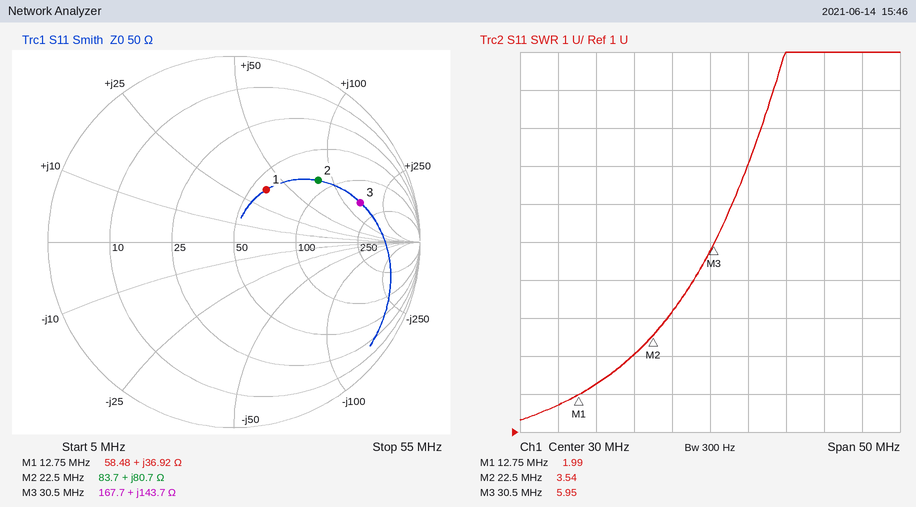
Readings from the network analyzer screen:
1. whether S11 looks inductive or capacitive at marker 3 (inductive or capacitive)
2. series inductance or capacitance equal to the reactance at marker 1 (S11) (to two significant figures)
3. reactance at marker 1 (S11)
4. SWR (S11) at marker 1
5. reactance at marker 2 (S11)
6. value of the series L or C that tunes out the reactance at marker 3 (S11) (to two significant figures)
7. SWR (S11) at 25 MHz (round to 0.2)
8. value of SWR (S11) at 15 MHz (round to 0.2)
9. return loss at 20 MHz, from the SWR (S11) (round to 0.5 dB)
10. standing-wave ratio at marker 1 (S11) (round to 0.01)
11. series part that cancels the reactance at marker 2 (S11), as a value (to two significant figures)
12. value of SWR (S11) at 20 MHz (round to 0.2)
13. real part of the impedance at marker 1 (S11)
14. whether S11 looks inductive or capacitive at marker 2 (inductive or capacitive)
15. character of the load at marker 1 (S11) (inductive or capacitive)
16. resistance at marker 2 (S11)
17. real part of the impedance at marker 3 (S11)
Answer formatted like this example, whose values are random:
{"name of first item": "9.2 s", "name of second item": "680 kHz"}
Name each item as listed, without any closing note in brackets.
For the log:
{"whether S11 looks inductive or capacitive at marker 3": "inductive", "series inductance or capacitance equal to the reactance at marker 1 (S11)": "460 nH", "reactance at marker 1": "+36.92 Ω", "SWR (S11) at marker 1": "1.99", "reactance at marker 2": "+80.7 Ω", "value of the series L or C that tunes out the reactance at marker 3 (S11)": "36 pF", "SWR (S11) at 25 MHz": "4.2", "value of SWR (S11) at 15 MHz": "2.2", "return loss at 20 MHz, from the SWR (S11)": "6.0 dB", "standing-wave ratio at marker 1 (S11)": "1.99", "series part that cancels the reactance at marker 2 (S11), as a value": "88 pF", "value of SWR (S11) at 20 MHz": "3.0", "real part of the impedance at marker 1": "58.48 Ω", "whether S11 looks inductive or capacitive at marker 2": "inductive", "character of the load at marker 1 (S11)": "inductive", "resistance at marker 2": "83.7 Ω", "real part of the impedance at marker 3": "167.7 Ω"}
